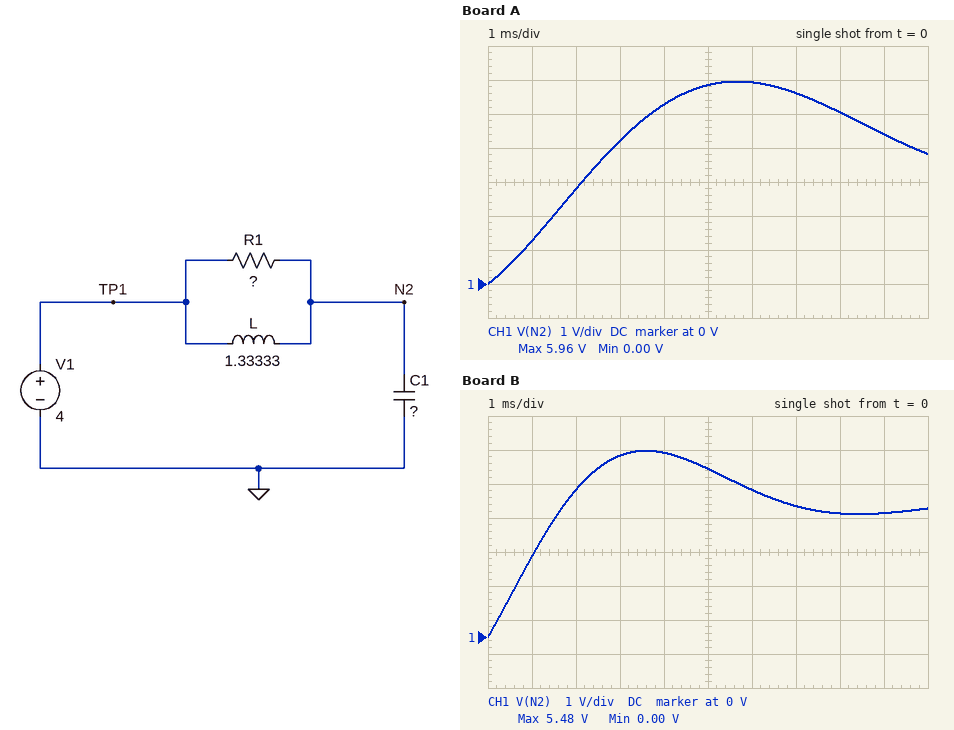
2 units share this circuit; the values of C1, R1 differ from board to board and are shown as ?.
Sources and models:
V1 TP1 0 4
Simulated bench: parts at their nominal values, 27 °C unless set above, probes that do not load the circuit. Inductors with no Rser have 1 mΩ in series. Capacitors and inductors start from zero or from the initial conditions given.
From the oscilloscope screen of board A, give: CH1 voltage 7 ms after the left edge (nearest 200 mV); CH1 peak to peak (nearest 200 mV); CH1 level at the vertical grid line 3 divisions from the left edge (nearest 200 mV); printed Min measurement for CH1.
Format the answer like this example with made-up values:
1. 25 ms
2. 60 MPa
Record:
1. 5.6 V
2. 6.0 V
3. 4.2 V
4. 0.00 V
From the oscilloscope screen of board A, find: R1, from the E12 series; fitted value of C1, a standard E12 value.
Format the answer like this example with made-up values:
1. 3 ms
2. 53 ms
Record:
1. 1.2 kΩ
2. 3.3 µF
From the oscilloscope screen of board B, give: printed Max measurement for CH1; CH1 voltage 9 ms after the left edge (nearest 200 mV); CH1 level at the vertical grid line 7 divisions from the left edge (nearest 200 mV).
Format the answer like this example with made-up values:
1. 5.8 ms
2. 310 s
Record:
1. 5.48 V
2. 3.6 V
3. 3.8 V
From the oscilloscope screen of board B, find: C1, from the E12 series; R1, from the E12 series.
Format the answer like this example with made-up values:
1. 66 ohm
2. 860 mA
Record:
1. 1.5 µF
2. 1.2 kΩ
